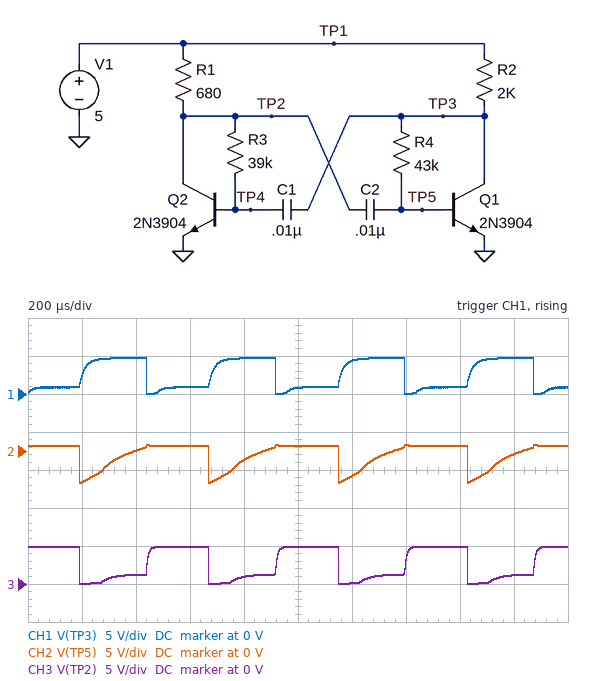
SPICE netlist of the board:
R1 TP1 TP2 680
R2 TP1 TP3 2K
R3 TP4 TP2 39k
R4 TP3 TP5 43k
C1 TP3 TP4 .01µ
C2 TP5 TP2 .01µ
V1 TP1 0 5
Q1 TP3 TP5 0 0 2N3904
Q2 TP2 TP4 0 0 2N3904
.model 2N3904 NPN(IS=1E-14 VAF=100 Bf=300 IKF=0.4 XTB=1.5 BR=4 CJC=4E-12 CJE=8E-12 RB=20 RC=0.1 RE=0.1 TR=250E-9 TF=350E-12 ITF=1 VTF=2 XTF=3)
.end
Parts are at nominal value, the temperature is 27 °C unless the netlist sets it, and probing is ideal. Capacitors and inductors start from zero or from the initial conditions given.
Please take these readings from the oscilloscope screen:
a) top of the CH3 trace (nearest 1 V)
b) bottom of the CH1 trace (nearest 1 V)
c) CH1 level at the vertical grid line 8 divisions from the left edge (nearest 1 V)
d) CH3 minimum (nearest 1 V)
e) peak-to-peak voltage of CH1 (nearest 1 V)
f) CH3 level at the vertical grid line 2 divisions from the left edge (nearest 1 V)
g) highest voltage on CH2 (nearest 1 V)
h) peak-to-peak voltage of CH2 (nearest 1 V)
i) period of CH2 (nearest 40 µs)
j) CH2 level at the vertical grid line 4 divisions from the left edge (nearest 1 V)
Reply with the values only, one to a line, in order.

5 V
0 V
1 V
0 V
5 V
1 V
1 V
5 V
480 µs
-1 V
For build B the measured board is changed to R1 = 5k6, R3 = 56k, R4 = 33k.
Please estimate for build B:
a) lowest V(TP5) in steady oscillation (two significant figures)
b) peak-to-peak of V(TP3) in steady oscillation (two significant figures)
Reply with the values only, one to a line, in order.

-3.8 V
4.7 V
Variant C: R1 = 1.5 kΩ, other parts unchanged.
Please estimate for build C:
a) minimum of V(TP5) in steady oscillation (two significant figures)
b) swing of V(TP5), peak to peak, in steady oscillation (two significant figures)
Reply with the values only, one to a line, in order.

-4.1 V
4.9 V
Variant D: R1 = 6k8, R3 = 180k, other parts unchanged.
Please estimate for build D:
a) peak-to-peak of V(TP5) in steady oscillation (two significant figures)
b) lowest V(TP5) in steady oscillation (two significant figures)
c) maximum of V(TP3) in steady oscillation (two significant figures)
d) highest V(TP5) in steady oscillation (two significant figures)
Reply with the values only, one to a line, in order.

4.8 V
-4.1 V
4.8 V
710 mV
